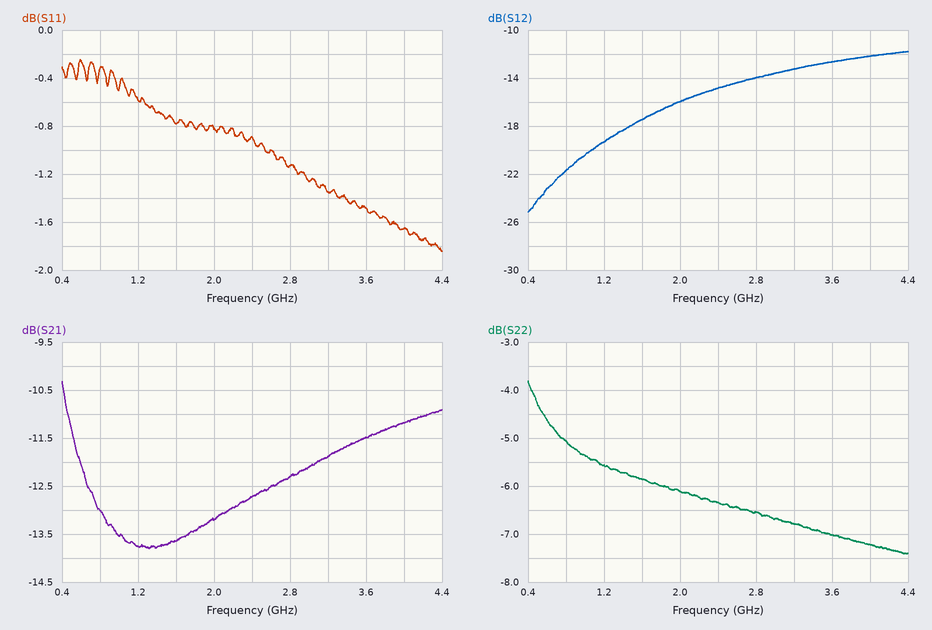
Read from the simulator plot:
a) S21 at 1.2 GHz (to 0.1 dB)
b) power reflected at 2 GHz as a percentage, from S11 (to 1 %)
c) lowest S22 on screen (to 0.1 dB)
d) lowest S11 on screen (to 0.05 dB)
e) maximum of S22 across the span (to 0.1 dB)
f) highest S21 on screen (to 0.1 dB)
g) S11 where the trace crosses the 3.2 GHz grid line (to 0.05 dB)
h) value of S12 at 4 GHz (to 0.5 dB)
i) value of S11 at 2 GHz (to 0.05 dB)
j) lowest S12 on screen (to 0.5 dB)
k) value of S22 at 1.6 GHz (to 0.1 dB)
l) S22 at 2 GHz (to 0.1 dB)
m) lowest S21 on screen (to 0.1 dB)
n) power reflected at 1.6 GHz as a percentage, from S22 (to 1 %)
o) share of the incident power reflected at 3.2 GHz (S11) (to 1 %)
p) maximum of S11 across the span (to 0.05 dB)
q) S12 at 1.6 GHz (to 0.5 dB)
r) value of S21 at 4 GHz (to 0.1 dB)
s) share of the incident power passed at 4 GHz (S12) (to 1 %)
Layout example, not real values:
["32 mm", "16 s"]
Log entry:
["-13.8 dB", "83 %", "-7.4 dB", "-1.85 dB", "-3.8 dB", "-10.3 dB", "-1.35 dB", "-12.0 dB", "-0.80 dB", "-25.0 dB", "-5.9 dB", "-6.1 dB", "-13.8 dB", "26 %", "73 %", "-0.25 dB", "-17.5 dB", "-11.2 dB", "6 %"]
